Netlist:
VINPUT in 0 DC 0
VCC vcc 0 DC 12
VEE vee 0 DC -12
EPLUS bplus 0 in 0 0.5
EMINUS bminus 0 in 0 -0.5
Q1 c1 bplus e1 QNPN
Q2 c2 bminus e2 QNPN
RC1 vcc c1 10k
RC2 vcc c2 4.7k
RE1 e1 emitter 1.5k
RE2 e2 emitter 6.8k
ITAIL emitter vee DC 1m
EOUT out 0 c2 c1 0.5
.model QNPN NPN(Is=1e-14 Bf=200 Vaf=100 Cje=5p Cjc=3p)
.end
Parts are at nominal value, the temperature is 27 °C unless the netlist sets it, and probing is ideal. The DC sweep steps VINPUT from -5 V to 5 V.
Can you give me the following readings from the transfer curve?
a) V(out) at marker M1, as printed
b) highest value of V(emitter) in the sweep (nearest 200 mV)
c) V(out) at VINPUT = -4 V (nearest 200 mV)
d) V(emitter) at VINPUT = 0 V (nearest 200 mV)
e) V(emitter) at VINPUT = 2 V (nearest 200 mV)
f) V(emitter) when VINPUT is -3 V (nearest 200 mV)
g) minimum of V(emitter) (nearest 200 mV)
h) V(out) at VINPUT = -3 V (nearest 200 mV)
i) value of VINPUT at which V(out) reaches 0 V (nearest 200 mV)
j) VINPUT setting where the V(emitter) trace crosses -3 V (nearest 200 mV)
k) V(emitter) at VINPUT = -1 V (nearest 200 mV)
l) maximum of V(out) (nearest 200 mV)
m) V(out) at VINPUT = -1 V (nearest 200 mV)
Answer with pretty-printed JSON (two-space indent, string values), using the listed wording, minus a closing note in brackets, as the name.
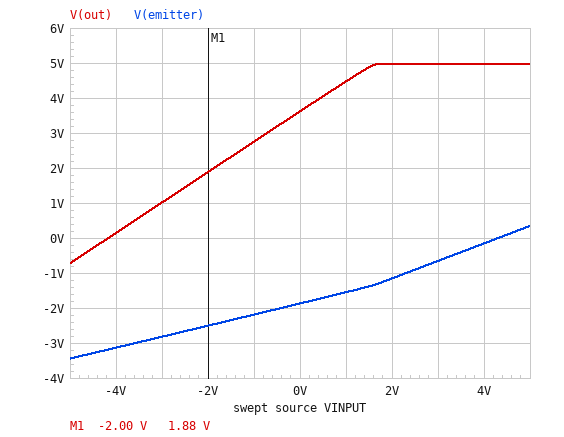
{
  "V(out) at marker M1, as printed": "1.88 V",
  "highest value of V(emitter) in the sweep": "400 mV",
  "V(out) at VINPUT = -4 V": "200 mV",
  "V(emitter) at VINPUT = 0 V": "-1.8 V",
  "V(emitter) at VINPUT = 2 V": "-1.2 V",
  "V(emitter) when VINPUT is -3 V": "-2.8 V",
  "minimum of V(emitter)": "-3.4 V",
  "V(out) at VINPUT = -3 V": "1.0 V",
  "value of VINPUT at which V(out) reaches 0 V": "-4.2 V",
  "VINPUT setting where the V(emitter) trace crosses -3 V": "-3.6 V",
  "V(emitter) at VINPUT = -1 V": "-2.2 V",
  "maximum of V(out)": "5.0 V",
  "V(out) at VINPUT = -1 V": "2.8 V"
}
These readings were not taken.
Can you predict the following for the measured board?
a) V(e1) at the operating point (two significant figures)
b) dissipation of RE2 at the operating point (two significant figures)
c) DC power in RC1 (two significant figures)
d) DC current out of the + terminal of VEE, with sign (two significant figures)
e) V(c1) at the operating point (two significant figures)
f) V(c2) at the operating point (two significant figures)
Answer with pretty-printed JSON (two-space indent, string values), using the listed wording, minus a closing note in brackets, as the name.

{
  "V(e1) at the operating point": "-650 mV",
  "dissipation of RE2 at the operating point": "230 µW",
  "DC power in RC1": "6.6 mW",
  "DC current out of the + terminal of VEE, with sign": "-1.0 mA",
  "V(c1) at the operating point": "3.9 V",
  "V(c2) at the operating point": "11 V"
}
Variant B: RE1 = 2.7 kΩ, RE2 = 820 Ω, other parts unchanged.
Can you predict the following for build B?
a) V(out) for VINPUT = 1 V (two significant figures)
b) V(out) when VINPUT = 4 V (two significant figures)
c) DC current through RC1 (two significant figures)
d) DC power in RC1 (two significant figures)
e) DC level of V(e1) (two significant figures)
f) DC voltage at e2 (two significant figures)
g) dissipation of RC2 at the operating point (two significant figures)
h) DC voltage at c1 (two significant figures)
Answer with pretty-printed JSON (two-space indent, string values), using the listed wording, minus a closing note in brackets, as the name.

{
  "V(out) for VINPUT = 1 V": "1.4 V",
  "V(out) when VINPUT = 4 V": "5.0 V",
  "DC current through RC1": "240 µA",
  "DC power in RC1": "580 µW",
  "DC level of V(e1)": "-620 mV",
  "DC voltage at e2": "-650 mV",
  "dissipation of RC2 at the operating point": "2.7 mW",
  "DC voltage at c1": "9.6 V"
}
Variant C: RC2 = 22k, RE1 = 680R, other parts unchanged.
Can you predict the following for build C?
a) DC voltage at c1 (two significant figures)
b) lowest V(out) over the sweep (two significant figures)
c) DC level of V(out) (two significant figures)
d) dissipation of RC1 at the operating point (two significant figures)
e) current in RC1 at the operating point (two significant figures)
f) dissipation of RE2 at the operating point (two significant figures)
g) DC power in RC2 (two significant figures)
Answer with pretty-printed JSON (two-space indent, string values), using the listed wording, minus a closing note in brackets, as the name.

{
  "DC voltage at c1": "3.0 V",
  "lowest V(out) over the sweep": "-3.8 V",
  "DC level of V(out)": "3.4 V",
  "dissipation of RC1 at the operating point": "8.0 mW",
  "current in RC1 at the operating point": "900 µA",
  "dissipation of RE2 at the operating point": "66 µW",
  "DC power in RC2": "210 µW"
}
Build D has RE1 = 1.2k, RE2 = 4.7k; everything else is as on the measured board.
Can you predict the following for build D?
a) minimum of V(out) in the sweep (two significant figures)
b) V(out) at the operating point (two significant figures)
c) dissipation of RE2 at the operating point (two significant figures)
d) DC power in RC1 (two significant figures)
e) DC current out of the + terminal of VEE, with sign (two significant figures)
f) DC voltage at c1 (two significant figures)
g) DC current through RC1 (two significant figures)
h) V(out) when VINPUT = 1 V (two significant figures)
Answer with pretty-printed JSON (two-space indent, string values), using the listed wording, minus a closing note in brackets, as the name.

{
  "minimum of V(out) in the sweep": "-2.3 V",
  "V(out) at the operating point": "3.4 V",
  "dissipation of RE2 at the operating point": "210 µW",
  "DC power in RC1": "6.2 mW",
  "DC current out of the + terminal of VEE, with sign": "-1.0 mA",
  "DC voltage at c1": "4.1 V",
  "DC current through RC1": "790 µA",
  "V(out) when VINPUT = 1 V": "4.6 V"
}
